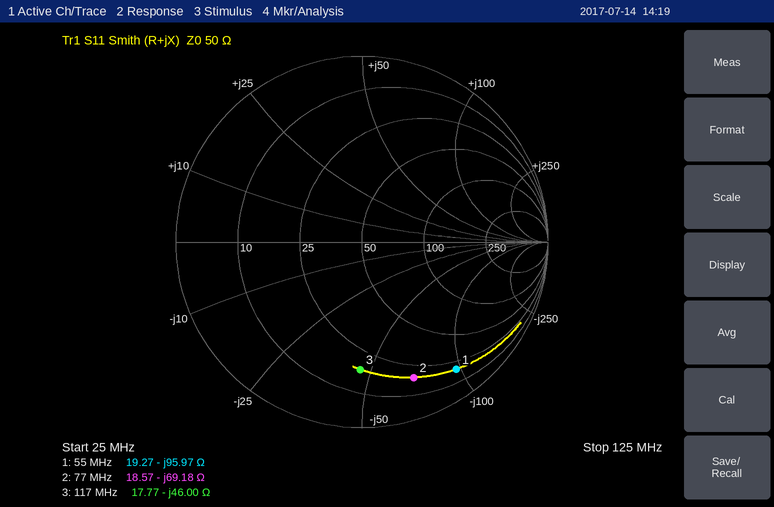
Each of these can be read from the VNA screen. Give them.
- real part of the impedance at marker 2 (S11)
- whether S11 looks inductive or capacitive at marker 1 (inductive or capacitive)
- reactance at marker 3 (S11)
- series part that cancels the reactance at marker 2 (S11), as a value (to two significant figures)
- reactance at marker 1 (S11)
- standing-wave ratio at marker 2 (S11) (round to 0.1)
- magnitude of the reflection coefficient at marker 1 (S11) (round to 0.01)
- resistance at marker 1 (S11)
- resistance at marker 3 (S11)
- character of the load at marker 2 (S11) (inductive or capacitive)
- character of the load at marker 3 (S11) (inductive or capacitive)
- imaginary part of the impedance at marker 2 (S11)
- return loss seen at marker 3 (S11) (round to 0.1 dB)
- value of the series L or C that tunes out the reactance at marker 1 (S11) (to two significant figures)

18.57 Ω
capacitive
-46.00 Ω
140 nH
-95.97 Ω
8.1
0.85
19.27 Ω
17.77 Ω
capacitive
capacitive
-69.18 Ω
3.3 dB
280 nH
